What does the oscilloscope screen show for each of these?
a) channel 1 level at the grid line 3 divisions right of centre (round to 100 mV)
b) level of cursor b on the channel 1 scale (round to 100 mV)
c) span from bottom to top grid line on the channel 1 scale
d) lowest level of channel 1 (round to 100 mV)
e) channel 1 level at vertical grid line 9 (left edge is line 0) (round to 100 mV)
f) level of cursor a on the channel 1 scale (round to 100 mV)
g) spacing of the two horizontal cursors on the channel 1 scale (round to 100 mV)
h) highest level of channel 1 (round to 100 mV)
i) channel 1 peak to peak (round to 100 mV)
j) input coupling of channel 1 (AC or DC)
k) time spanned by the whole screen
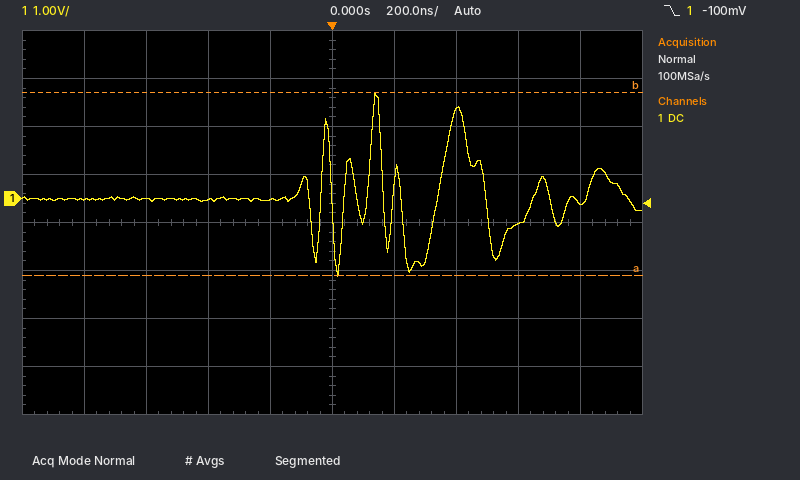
-500 mV
2.2 V
8 V
-1.6 V
-100 mV
-1.6 V
3.8 V
2.2 V
3.8 V
DC
2 µs
